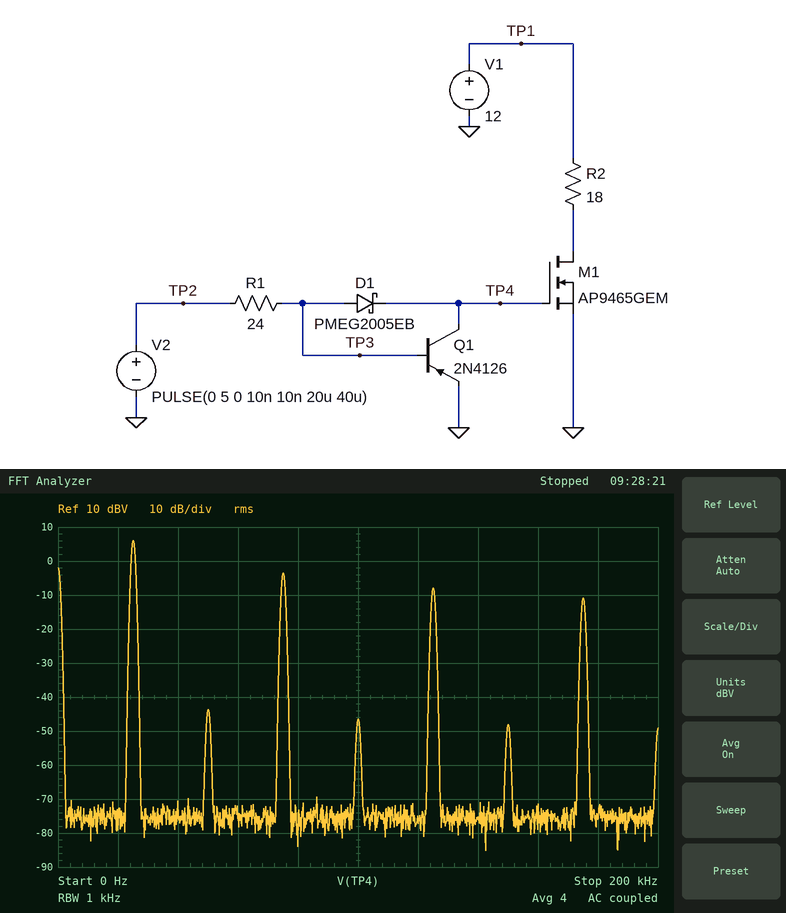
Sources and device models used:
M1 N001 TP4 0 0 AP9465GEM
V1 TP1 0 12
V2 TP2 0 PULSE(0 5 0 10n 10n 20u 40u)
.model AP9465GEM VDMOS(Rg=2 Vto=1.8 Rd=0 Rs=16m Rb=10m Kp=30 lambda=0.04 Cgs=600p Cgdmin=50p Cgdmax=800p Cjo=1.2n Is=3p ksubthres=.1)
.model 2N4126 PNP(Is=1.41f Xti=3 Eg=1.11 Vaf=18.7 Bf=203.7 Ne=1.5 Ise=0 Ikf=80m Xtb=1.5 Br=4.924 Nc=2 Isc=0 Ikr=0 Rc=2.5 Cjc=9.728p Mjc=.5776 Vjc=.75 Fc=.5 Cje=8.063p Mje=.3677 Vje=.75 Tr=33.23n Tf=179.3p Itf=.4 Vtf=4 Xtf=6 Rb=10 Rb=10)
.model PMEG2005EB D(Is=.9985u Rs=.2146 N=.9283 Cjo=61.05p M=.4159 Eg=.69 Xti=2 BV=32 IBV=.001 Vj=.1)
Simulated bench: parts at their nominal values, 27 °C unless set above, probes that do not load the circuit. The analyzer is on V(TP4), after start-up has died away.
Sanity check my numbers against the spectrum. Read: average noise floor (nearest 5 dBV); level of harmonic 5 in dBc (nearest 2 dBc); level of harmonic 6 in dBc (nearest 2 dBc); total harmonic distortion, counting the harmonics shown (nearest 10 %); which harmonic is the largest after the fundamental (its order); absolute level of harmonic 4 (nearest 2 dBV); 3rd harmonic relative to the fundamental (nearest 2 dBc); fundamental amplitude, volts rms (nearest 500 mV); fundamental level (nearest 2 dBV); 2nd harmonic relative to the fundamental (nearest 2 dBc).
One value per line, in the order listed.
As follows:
-75 dBV
-14 dBc
-54 dBc
40 %
3
-46 dBV
-10 dBc
2.0 V
6 dBV
-50 dBc
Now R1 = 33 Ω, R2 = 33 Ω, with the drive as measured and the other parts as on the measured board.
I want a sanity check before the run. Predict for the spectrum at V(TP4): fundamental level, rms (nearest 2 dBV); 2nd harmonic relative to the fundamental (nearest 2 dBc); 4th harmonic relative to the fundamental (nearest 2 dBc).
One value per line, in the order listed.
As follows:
6 dBV
-48 dBc
-50 dBc
